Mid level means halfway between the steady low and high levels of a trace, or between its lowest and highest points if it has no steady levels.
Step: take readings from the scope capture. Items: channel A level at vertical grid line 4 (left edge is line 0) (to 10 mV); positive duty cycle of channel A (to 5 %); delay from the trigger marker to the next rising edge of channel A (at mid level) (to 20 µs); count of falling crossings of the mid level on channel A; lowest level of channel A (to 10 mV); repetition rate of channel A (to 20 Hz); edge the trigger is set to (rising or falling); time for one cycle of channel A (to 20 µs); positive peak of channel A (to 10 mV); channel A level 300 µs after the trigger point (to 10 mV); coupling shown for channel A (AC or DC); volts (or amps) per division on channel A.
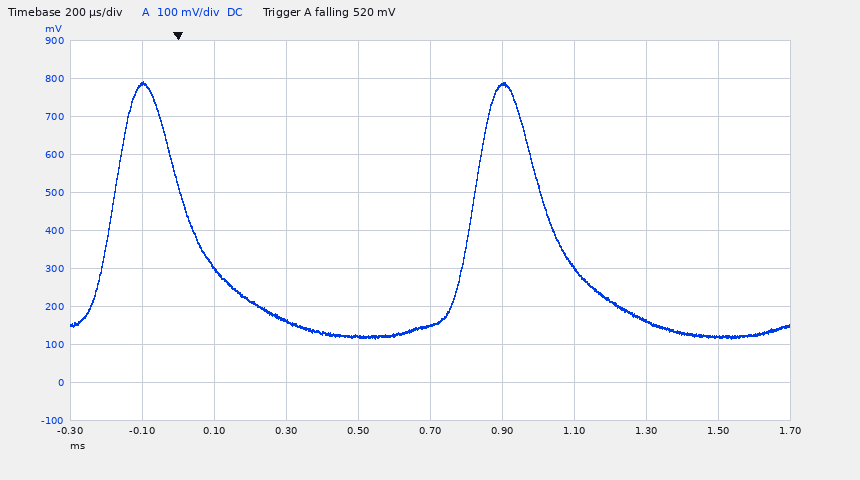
120 mV
20 %
820 µs
2
120 mV
1.00 kHz
falling
1.00 ms
790 mV
160 mV
DC
100 mV
